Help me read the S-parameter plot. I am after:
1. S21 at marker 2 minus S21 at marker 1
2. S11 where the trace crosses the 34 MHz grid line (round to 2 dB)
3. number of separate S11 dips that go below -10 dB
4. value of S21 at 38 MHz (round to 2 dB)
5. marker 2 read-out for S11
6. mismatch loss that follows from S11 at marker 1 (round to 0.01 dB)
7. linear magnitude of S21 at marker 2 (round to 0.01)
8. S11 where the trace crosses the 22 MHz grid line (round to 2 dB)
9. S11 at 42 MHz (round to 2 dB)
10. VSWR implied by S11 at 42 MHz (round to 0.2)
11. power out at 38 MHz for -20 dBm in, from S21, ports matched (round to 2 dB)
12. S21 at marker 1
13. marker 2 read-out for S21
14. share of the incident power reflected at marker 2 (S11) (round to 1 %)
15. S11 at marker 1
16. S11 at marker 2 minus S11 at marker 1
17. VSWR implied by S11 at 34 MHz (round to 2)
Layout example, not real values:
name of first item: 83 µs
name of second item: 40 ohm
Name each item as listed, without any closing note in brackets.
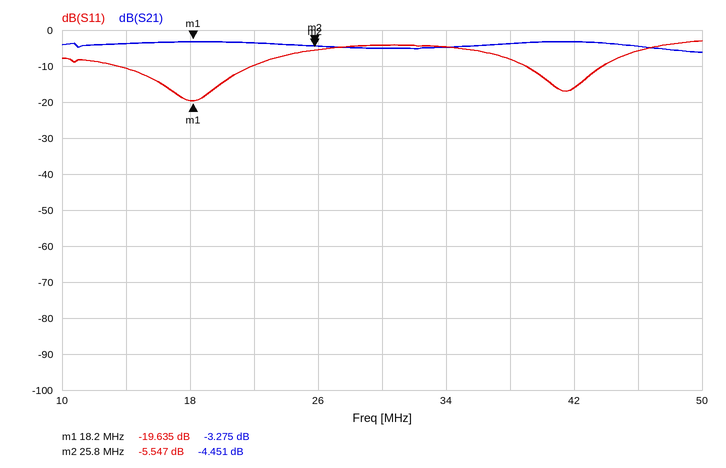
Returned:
S21 at marker 2 minus S21 at marker 1: -1.176 dB
S11 where the trace crosses the 34 MHz grid line: -4 dB
number of separate S11 dips that go below -10 dB: 2
value of S21 at 38 MHz: -4 dB
marker 2 read-out for S11: -5.547 dB
mismatch loss that follows from S11 at marker 1: 0.05 dB
linear magnitude of S21 at marker 2: 0.60
S11 where the trace crosses the 22 MHz grid line: -10 dB
S11 at 42 MHz: -16 dB
VSWR implied by S11 at 42 MHz: 1.4
power out at 38 MHz for -20 dBm in, from S21, ports matched: -24 dBm
S21 at marker 1: -3.275 dB
marker 2 read-out for S21: -4.451 dB
share of the incident power reflected at marker 2 (S11): 28 %
S11 at marker 1: -19.635 dB
S11 at marker 2 minus S11 at marker 1: 14.088 dB
VSWR implied by S11 at 34 MHz: 4
